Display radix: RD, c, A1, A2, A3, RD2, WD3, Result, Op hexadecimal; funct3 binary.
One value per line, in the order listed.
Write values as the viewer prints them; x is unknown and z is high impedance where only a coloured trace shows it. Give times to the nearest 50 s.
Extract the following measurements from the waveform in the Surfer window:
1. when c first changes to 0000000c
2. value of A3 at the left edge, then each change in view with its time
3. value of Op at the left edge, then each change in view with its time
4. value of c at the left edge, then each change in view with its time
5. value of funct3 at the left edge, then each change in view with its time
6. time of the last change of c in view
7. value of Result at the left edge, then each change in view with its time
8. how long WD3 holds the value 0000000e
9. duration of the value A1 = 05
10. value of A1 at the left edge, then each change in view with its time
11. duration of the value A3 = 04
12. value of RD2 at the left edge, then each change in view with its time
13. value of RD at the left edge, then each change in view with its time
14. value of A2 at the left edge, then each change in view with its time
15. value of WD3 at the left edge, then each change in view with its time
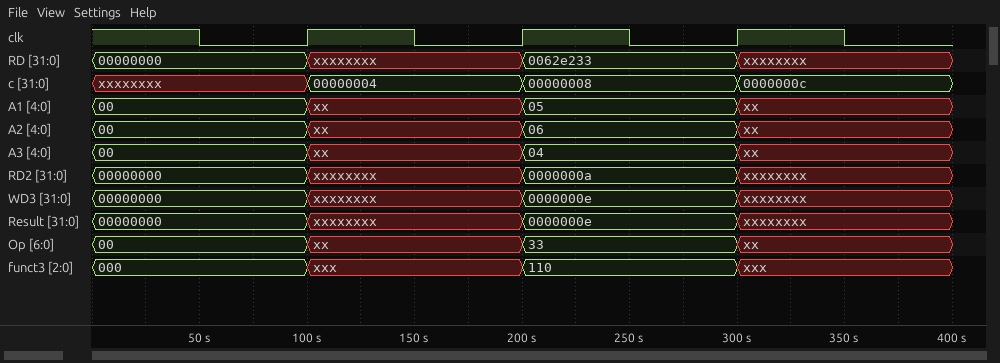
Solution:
300 s
00, xx at 100 s, 04 at 200 s, xx at 300 s
00, xx at 100 s, 33 at 200 s, xx at 300 s
xxxxxxxx, 00000004 at 100 s, 00000008 at 200 s, 0000000c at 300 s
000, xxx at 100 s, 110 at 200 s, xxx at 300 s
300 s
00000000, xxxxxxxx at 100 s, 0000000e at 200 s, xxxxxxxx at 300 s
100 s
100 s
00, xx at 100 s, 05 at 200 s, xx at 300 s
100 s
00000000, xxxxxxxx at 100 s, 0000000a at 200 s, xxxxxxxx at 300 s
00000000, xxxxxxxx at 100 s, 0062e233 at 200 s, xxxxxxxx at 300 s
00, xx at 100 s, 06 at 200 s, xx at 300 s
00000000, xxxxxxxx at 100 s, 0000000e at 200 s, xxxxxxxx at 300 s
